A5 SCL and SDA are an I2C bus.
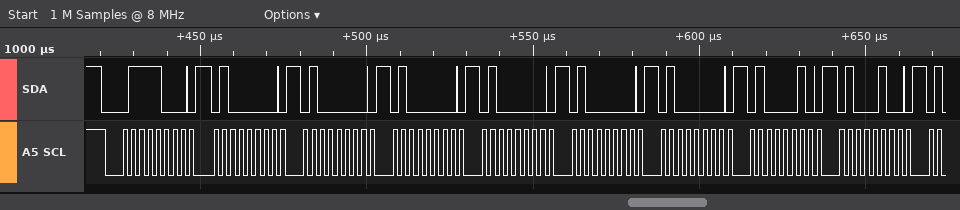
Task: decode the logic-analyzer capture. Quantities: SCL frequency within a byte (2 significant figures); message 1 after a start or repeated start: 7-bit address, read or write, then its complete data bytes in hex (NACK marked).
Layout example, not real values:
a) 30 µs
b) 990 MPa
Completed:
a) 400 kHz
b) 0x3C write: 40 40 40 40 40 40 42 44
